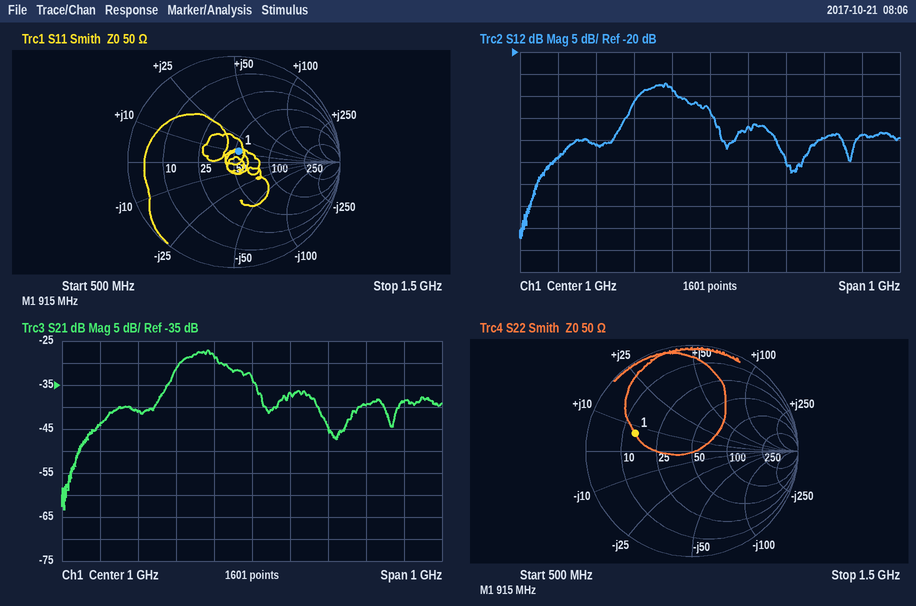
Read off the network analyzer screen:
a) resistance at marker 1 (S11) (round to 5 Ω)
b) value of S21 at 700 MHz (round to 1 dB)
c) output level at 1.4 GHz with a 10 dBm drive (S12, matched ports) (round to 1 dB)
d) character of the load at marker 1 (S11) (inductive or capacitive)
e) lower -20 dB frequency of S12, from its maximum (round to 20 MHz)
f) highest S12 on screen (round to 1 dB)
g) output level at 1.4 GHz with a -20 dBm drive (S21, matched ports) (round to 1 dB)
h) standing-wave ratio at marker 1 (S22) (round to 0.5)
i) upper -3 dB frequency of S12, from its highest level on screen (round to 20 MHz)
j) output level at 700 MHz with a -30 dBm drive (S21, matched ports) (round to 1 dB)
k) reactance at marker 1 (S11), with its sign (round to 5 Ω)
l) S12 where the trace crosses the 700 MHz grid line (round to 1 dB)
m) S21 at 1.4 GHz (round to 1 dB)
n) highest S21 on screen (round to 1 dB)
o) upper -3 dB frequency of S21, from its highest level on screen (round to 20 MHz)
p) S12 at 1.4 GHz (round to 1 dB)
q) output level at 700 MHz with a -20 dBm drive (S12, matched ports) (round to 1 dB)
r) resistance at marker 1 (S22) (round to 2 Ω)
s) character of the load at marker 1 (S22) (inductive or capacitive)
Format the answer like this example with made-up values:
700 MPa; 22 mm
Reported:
55 Ω; -41 dB; -29 dBm; inductive; 560 MHz; -27 dB; -59 dBm; 3.5; 920 MHz; -71 dBm; +10 Ω; -41 dB; -39 dB; -27 dB; 920 MHz; -39 dB; -61 dBm; 14 Ω; inductive
